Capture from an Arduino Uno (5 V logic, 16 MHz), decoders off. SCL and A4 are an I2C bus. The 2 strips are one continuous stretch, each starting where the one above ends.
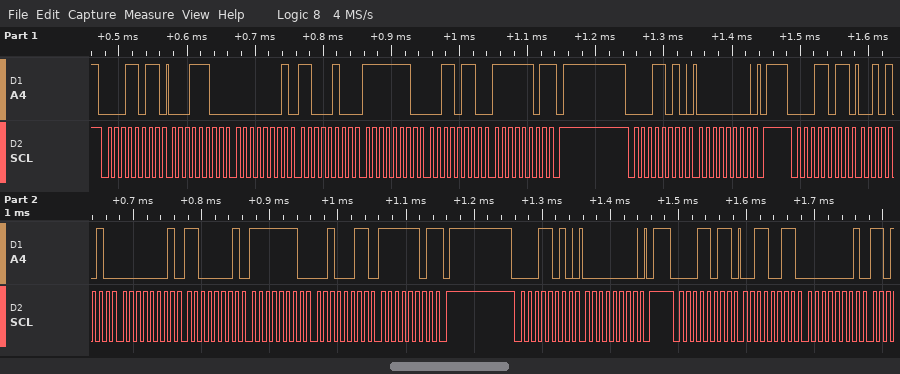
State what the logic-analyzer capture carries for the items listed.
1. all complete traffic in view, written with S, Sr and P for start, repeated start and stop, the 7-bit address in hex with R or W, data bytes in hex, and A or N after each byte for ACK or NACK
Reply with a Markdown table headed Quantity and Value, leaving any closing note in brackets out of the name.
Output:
| Quantity | Value |
|---|---|
| all complete traffic in view, written with S, Sr and P for start, repeated start and stop, the 7-bit address in hex with R or W, data bytes in hex, and A or N after each byte for ACK or NACK | S 0DR A 1C A 01 A C4 A FE A 36 A FD N P S 0DW A 00 A P S 0DR A 2A A 01 A C1 A FE A 23 A FD N P S 0DW A 00 A P S 0DR A 33 A 01 A |
